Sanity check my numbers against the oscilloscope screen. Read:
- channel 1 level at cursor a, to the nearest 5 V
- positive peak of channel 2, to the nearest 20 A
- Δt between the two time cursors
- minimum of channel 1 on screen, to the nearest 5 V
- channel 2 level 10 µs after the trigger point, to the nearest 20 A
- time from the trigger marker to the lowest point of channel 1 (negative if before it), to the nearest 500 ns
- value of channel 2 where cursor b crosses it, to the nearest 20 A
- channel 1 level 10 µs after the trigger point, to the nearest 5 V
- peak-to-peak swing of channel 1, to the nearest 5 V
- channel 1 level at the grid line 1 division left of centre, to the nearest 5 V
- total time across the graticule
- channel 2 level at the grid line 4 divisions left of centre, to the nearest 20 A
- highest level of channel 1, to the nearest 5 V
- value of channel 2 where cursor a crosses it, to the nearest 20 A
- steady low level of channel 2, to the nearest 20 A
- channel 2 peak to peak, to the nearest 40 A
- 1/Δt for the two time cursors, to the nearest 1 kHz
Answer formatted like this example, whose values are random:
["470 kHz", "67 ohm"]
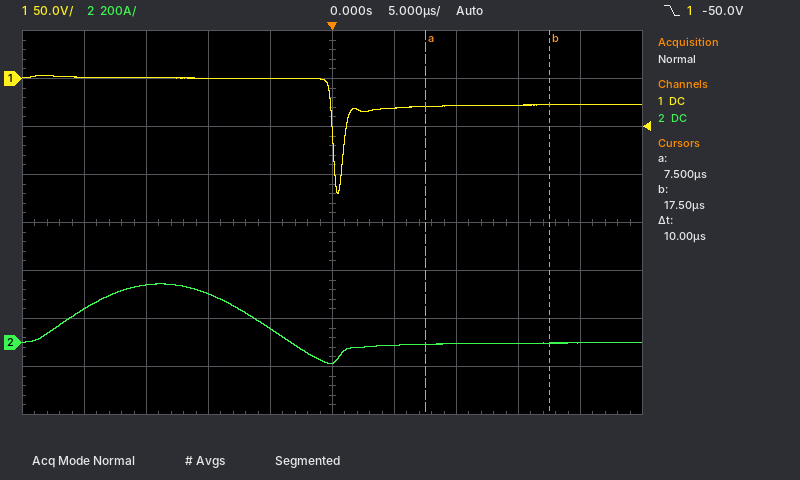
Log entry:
["-30 V", "240 A", "10 µs", "-120 V", "0 A", "+500 ns", "0 A", "-30 V", "125 V", "0 V", "50 µs", "140 A", "5 V", "0 A", "0 A", "320 A", "100 kHz"]
